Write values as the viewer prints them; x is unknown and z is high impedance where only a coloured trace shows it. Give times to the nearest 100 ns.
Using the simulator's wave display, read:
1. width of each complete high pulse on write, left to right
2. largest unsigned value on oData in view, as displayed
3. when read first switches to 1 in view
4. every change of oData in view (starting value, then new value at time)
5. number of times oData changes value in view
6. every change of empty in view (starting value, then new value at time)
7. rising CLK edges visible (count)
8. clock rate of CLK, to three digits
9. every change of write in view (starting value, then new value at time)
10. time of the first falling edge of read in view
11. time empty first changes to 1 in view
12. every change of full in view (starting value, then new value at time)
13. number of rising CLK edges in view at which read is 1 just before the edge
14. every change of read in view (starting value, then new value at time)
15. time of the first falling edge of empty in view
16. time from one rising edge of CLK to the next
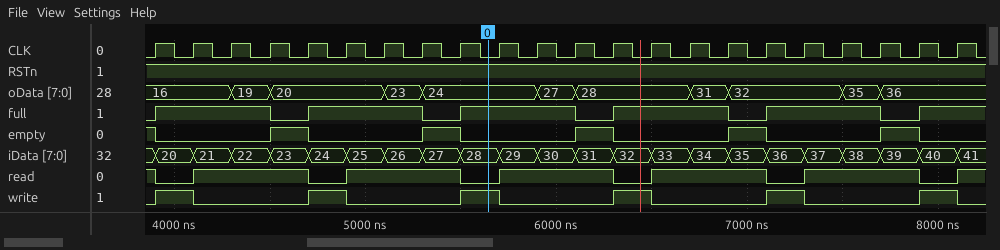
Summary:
200 ns, 200 ns, 200 ns, 200 ns, 200 ns, 200 ns
36
4100 ns
16, 19 at 4300 ns, 20 at 4500 ns, 23 at 5100 ns, 24 at 5300 ns, 27 at 5900 ns, 28 at 6100 ns, 31 at 6700 ns, 32 at 6900 ns, 35 at 7500 ns, 36 at 7700 ns
10
1, 0 at 3900 ns, 1 at 4500 ns, 0 at 4700 ns, 1 at 5300 ns, 0 at 5500 ns, 1 at 6100 ns, 0 at 6300 ns, 1 at 6900 ns, 0 at 7100 ns, 1 at 7700 ns, 0 at 7900 ns
22
5.00 MHz
0, 1 at 3900 ns, 0 at 4100 ns, 1 at 4700 ns, 0 at 4900 ns, 1 at 5500 ns, 0 at 5700 ns, 1 at 6300 ns, 0 at 6500 ns, 1 at 7100 ns, 0 at 7300 ns, 1 at 7900 ns, 0 at 8100 ns
3900 ns
4500 ns
0, 1 at 3900 ns, 0 at 4500 ns, 1 at 4700 ns, 0 at 5300 ns, 1 at 5500 ns, 0 at 6100 ns, 1 at 6300 ns, 0 at 6900 ns, 1 at 7100 ns, 0 at 7700 ns, 1 at 7900 ns
16
1, 0 at 3900 ns, 1 at 4100 ns, 0 at 4700 ns, 1 at 4900 ns, 0 at 5500 ns, 1 at 5700 ns, 0 at 6300 ns, 1 at 6500 ns, 0 at 7100 ns, 1 at 7300 ns, 0 at 7900 ns, 1 at 8100 ns
3900 ns
200 ns
